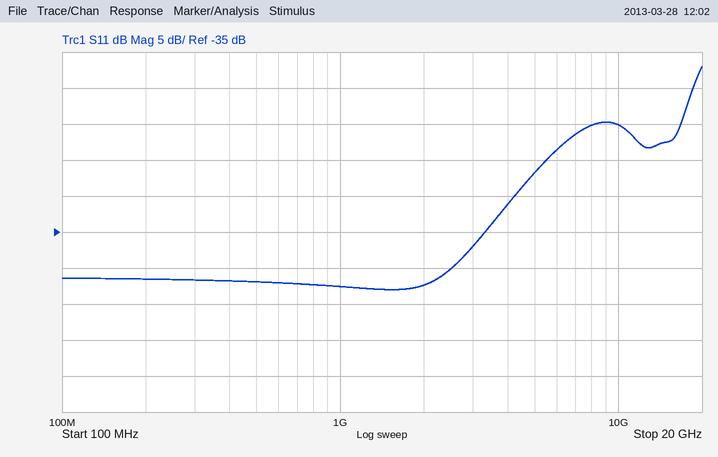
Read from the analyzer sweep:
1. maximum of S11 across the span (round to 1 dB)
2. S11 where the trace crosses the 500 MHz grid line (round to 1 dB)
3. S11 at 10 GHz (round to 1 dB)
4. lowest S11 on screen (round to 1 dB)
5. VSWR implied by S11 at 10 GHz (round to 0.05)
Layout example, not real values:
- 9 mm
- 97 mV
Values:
- -12 dB
- -42 dB
- -20 dB
- -43 dB
- 1.20
